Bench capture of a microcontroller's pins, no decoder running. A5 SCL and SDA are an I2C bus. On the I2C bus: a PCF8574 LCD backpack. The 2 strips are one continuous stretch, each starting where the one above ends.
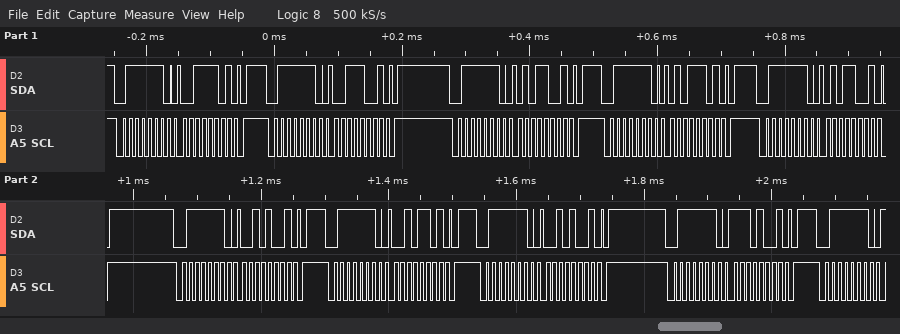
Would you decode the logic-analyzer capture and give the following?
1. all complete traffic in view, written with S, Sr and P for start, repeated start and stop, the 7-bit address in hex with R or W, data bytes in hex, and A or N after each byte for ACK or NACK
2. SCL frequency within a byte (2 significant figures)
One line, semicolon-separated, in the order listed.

S 3FW A 3D A P S 3FW A 39 A P S 3FW A 59 A P S 3FW A 5D A P S 3FW A 59 A P S 3FW A 29 A P S 3FW A 2D A P S 3FW A 29 A P S 3FW A E9 A P S 3FW A; 100 kHz
